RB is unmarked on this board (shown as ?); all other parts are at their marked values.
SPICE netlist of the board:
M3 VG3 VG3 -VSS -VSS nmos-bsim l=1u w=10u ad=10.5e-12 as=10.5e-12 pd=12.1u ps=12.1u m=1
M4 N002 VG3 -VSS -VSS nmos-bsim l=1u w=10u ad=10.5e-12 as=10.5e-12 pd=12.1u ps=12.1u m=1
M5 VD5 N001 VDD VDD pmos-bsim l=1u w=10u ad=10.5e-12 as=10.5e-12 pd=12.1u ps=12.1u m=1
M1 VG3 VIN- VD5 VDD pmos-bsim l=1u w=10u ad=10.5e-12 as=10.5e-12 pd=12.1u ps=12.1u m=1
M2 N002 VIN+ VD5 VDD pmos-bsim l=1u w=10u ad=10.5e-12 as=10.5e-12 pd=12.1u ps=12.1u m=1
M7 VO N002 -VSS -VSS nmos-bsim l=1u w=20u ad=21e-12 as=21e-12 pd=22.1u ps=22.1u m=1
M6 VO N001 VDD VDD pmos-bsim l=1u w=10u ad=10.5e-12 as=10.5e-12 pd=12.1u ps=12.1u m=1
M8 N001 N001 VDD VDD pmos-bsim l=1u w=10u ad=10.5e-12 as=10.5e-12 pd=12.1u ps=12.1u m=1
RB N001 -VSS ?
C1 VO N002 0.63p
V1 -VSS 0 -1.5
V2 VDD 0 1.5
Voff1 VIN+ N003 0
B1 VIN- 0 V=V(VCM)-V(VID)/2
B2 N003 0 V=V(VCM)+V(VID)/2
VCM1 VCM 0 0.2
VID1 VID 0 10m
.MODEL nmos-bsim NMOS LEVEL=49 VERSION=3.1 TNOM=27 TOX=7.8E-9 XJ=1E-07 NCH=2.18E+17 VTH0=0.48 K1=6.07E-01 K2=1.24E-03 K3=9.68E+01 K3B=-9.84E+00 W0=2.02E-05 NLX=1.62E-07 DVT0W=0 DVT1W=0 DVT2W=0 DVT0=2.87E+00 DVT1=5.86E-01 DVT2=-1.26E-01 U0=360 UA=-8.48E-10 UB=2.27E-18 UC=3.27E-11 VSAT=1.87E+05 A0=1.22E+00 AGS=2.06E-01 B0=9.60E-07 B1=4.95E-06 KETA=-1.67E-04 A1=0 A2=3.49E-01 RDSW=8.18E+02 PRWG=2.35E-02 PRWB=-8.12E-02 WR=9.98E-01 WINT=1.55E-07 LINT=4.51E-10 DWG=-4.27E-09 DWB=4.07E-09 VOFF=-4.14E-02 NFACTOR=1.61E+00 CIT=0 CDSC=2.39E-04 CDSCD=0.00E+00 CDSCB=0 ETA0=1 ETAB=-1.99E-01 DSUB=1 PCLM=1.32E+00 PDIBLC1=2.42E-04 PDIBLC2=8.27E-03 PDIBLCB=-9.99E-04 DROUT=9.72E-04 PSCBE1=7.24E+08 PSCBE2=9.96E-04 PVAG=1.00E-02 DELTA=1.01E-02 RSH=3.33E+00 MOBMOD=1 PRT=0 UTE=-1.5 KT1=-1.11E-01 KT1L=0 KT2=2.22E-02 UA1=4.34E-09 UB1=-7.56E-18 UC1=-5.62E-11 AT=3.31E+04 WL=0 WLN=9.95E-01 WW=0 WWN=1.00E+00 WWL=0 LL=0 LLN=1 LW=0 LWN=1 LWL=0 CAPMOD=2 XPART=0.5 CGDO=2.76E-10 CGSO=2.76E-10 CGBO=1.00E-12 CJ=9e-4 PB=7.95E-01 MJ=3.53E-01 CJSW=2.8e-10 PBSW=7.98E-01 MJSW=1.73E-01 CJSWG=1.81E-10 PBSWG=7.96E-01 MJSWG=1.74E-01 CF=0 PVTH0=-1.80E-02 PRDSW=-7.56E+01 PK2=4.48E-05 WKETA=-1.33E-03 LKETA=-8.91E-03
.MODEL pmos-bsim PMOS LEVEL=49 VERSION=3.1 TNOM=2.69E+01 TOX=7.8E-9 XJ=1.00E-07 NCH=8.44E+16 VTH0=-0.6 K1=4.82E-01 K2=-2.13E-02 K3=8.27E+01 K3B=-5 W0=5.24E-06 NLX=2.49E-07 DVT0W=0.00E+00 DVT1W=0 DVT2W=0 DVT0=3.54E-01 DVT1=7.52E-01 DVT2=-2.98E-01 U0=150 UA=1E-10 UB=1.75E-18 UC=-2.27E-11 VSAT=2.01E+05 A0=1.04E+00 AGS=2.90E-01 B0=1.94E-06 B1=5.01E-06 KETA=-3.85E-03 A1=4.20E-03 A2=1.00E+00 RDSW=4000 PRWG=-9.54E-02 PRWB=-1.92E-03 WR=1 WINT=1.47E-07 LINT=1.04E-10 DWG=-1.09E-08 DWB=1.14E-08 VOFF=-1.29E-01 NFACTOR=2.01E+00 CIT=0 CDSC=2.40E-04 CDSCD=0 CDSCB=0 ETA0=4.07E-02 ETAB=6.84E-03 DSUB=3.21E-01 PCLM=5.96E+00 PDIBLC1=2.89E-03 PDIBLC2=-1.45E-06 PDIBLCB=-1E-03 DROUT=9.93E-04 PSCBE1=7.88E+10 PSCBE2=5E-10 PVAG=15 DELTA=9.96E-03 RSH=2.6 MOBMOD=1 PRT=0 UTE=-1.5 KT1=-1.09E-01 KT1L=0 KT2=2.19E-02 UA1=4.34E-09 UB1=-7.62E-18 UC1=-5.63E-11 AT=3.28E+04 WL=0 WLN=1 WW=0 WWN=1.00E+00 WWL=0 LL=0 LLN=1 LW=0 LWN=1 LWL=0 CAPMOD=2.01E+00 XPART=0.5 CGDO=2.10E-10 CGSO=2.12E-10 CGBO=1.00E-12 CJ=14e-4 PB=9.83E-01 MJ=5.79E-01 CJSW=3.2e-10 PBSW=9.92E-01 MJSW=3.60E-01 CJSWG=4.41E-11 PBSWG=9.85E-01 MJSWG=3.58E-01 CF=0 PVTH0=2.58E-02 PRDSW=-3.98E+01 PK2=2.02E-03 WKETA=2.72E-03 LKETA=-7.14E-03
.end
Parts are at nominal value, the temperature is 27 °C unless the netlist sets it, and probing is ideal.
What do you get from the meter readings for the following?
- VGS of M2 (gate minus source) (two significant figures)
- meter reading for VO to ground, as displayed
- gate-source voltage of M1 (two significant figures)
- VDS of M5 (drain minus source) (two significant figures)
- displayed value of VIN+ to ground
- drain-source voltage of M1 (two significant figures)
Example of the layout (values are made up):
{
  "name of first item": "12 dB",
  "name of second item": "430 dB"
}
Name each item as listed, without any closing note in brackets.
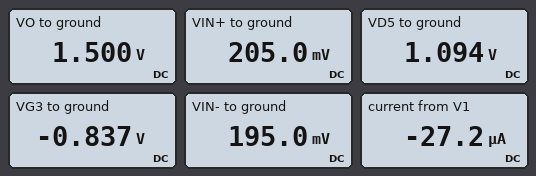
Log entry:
{
  "VGS of M2 (gate minus source)": "-890 mV",
  "meter reading for VO to ground, as displayed": "1.500 V",
  "gate-source voltage of M1": "-900 mV",
  "VDS of M5 (drain minus source)": "-410 mV",
  "displayed value of VIN+ to ground": "205.0 mV",
  "drain-source voltage of M1": "-1.9 V"
}
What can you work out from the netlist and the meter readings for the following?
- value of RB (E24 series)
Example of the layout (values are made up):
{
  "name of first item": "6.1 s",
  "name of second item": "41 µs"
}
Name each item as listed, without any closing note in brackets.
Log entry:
{
  "value of RB": "150 kΩ"
}
